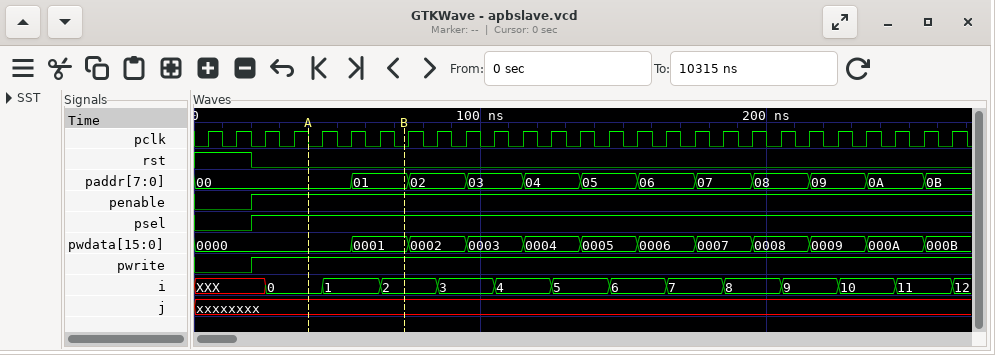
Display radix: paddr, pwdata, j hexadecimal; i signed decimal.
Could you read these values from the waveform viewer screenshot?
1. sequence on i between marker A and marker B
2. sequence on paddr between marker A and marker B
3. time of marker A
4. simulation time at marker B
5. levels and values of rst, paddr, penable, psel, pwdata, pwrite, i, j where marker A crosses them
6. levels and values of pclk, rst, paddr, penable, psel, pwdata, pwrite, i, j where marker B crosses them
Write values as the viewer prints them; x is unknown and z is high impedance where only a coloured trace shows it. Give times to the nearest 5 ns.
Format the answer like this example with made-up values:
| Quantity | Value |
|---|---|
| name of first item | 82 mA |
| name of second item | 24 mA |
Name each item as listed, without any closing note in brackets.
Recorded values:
| Quantity | Value |
|---|---|
| sequence on i between marker A and marker B | 0, 1, 2 |
| sequence on paddr between marker A and marker B | 00, 01 |
| time of marker A | 40 ns |
| simulation time at marker B | 75 ns |
| levels and values of rst, paddr, penable, psel, pwdata, pwrite, i, j where marker A crosses them | rst=0, paddr=00, penable=1, psel=1, pwdata=0000, pwrite=1, i=0, j=xxxxxxxx |
| levels and values of pclk, rst, paddr, penable, psel, pwdata, pwrite, i, j where marker B crosses them | pclk=0, rst=0, paddr=01, penable=1, psel=1, pwdata=0001, pwrite=1, i=2, j=xxxxxxxx |
